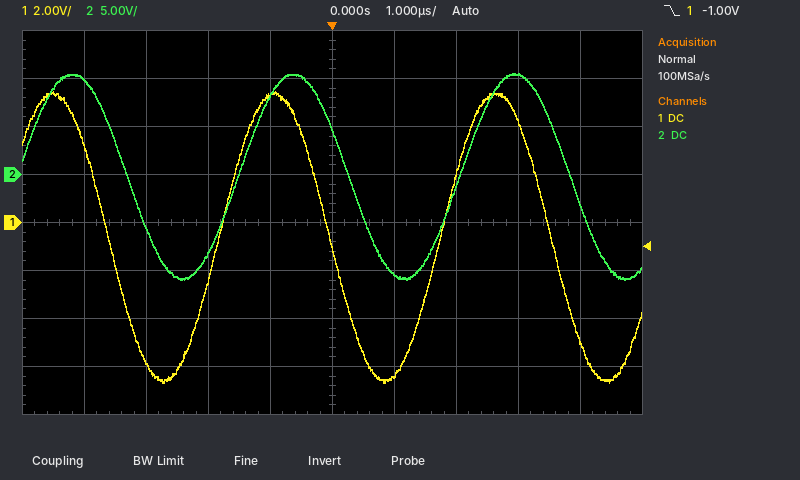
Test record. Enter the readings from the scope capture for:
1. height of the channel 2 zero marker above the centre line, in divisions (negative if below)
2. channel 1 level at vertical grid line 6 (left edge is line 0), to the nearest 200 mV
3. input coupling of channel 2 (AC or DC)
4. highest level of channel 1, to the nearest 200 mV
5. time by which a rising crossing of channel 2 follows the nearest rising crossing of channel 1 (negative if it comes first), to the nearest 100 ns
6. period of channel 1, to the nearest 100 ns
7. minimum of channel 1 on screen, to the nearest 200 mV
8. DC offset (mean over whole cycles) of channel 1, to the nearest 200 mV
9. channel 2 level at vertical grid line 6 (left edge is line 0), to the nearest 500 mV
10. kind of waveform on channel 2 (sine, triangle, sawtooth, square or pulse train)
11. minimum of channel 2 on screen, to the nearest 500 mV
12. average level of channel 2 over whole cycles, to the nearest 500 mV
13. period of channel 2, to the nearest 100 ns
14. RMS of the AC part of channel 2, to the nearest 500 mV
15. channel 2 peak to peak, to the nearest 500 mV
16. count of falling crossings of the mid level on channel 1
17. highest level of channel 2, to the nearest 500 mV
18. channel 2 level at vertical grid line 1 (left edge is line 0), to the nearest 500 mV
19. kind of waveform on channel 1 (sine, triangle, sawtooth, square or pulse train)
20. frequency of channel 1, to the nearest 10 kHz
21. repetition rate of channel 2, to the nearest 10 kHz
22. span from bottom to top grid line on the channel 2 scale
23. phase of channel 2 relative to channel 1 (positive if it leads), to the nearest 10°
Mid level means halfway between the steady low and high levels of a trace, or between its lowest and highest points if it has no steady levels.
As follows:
+1.0 div
-6.4 V
DC
5.4 V
+300 ns
3.6 µs
-6.6 V
-600 mV
-10.5 V
sine
-11.0 V
0.0 V
3.6 µs
7.5 V
21.5 V
3
10.5 V
10.0 V
sine
280 kHz
280 kHz
40 V
-30°
